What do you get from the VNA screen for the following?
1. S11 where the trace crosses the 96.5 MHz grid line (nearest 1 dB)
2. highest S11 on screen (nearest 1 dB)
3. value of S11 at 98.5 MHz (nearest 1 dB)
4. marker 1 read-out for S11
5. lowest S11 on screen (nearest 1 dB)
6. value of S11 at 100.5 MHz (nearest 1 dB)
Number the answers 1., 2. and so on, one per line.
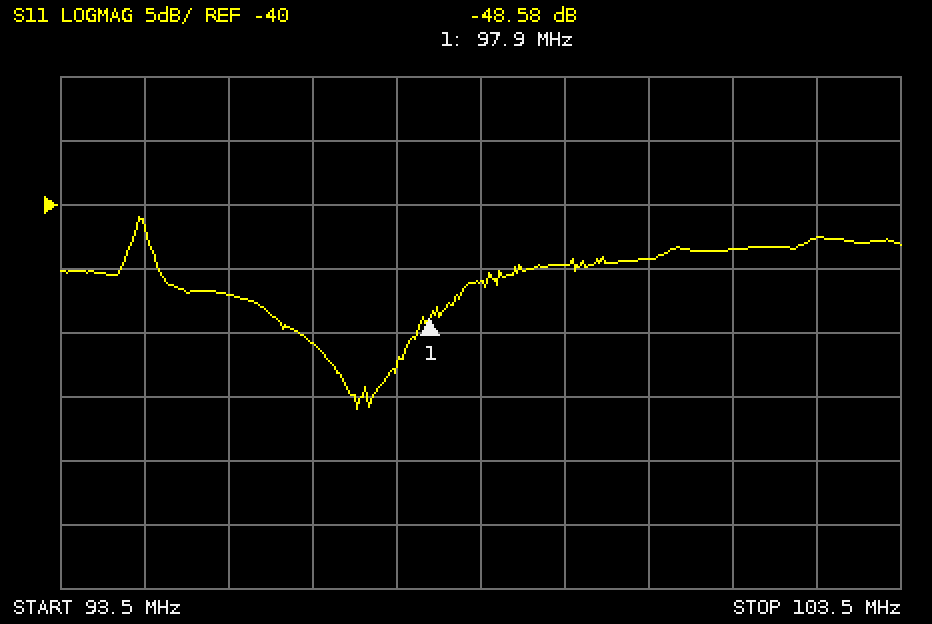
1. -51 dB
2. -41 dB
3. -46 dB
4. -48.58 dB
5. -56 dB
6. -44 dB
